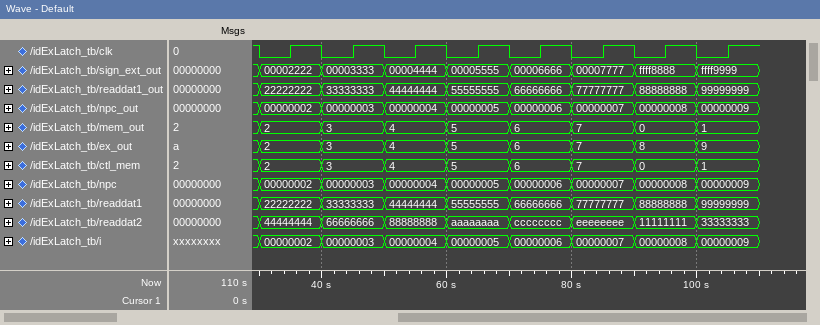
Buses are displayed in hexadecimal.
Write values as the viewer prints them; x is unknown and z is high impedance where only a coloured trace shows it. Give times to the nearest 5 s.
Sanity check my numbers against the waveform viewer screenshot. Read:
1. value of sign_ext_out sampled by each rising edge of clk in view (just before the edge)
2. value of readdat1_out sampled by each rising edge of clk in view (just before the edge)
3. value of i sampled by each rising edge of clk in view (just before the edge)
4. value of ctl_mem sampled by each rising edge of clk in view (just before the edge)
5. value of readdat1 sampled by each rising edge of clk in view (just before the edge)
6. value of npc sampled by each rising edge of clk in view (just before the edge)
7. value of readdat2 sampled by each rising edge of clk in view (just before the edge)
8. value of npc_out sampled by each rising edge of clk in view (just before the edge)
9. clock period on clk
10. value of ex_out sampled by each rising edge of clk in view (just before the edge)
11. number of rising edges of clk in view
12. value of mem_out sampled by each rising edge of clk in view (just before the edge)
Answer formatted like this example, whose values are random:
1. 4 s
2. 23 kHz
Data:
1. 00002222, 00003333, 00004444, 00005555, 00006666, 00007777, ffff8888, ffff9999
2. 22222222, 33333333, 44444444, 55555555, 66666666, 77777777, 88888888, 99999999
3. 00000002, 00000003, 00000004, 00000005, 00000006, 00000007, 00000008, 00000009
4. 2, 3, 4, 5, 6, 7, 0, 1
5. 22222222, 33333333, 44444444, 55555555, 66666666, 77777777, 88888888, 99999999
6. 00000002, 00000003, 00000004, 00000005, 00000006, 00000007, 00000008, 00000009
7. 44444444, 66666666, 88888888, aaaaaaaa, cccccccc, eeeeeeee, 11111111, 33333333
8. 00000002, 00000003, 00000004, 00000005, 00000006, 00000007, 00000008, 00000009
9. 10 s
10. 2, 3, 4, 5, 6, 7, 8, 9
11. 8
12. 2, 3, 4, 5, 6, 7, 0, 1
